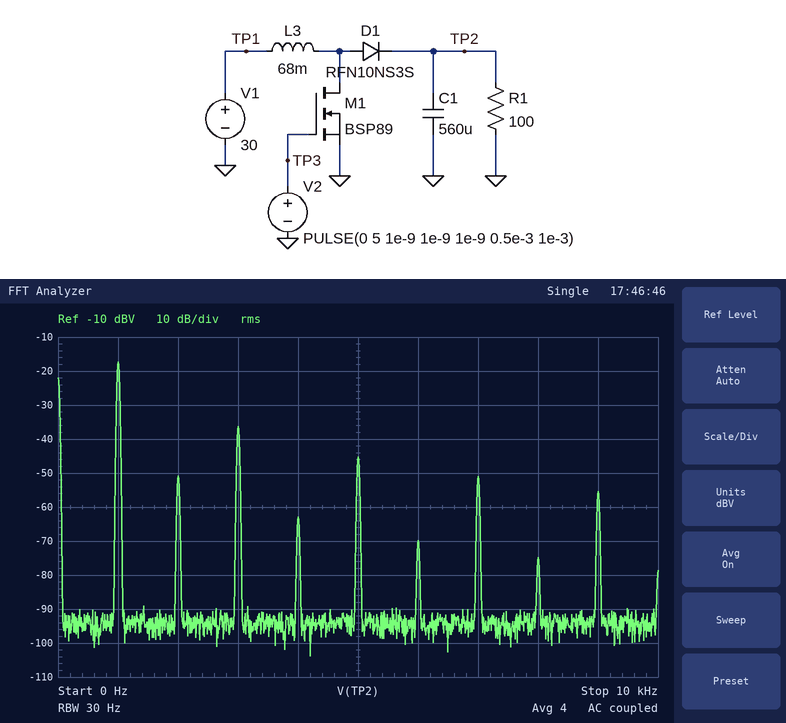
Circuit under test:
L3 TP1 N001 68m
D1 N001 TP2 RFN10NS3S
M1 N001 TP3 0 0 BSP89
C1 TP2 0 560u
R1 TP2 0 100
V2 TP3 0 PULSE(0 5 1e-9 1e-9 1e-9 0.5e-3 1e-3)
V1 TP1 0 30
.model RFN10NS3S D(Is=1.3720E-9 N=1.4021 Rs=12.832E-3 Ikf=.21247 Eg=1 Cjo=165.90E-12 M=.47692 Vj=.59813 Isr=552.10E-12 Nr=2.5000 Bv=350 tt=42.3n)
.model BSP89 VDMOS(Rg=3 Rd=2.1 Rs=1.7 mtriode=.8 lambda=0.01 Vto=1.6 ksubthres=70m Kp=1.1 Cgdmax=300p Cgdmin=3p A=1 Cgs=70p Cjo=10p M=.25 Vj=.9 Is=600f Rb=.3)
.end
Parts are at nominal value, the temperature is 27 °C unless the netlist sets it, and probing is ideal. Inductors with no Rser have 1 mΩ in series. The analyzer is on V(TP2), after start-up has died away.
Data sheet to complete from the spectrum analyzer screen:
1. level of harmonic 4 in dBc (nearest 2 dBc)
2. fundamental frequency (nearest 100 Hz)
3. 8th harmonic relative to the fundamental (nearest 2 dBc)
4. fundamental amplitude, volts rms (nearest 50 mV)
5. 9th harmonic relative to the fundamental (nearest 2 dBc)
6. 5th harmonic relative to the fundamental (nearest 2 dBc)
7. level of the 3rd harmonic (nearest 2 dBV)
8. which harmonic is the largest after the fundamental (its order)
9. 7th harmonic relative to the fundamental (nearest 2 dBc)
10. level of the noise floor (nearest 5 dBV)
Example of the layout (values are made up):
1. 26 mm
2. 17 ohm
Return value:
1. -46 dBc
2. 1.0 kHz
3. -58 dBc
4. 150 mV
5. -38 dBc
6. -28 dBc
7. -36 dBV
8. 3
9. -34 dBc
10. -95 dBV
